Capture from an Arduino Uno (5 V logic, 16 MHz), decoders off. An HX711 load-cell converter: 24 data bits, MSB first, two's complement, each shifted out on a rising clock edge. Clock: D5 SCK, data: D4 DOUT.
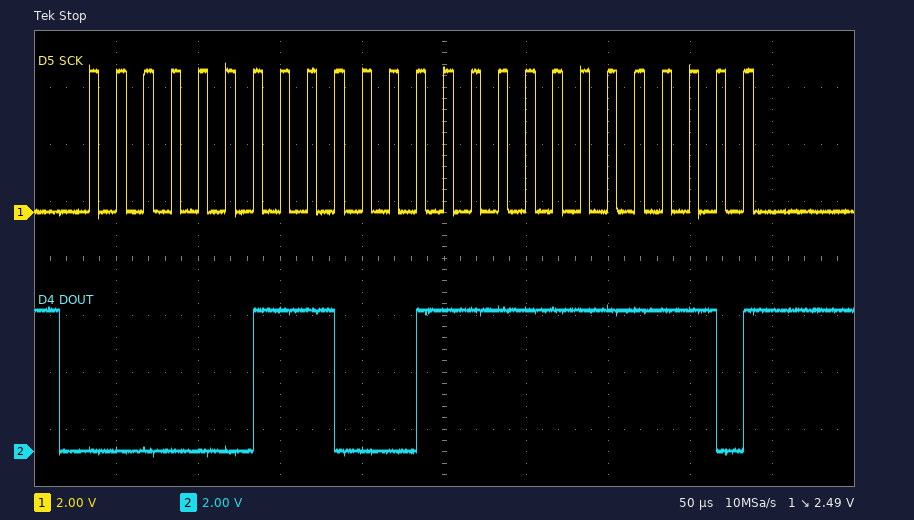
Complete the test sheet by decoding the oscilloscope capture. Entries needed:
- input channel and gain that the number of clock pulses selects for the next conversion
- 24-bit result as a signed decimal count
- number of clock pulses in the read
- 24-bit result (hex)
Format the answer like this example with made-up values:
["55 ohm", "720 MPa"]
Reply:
["channel A, gain 128", "233470", "25", "0x038FFE"]
